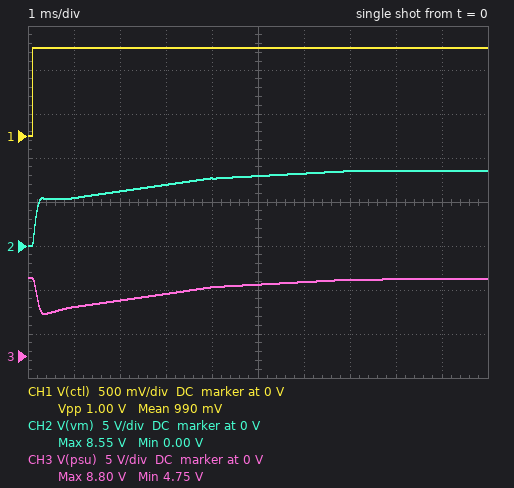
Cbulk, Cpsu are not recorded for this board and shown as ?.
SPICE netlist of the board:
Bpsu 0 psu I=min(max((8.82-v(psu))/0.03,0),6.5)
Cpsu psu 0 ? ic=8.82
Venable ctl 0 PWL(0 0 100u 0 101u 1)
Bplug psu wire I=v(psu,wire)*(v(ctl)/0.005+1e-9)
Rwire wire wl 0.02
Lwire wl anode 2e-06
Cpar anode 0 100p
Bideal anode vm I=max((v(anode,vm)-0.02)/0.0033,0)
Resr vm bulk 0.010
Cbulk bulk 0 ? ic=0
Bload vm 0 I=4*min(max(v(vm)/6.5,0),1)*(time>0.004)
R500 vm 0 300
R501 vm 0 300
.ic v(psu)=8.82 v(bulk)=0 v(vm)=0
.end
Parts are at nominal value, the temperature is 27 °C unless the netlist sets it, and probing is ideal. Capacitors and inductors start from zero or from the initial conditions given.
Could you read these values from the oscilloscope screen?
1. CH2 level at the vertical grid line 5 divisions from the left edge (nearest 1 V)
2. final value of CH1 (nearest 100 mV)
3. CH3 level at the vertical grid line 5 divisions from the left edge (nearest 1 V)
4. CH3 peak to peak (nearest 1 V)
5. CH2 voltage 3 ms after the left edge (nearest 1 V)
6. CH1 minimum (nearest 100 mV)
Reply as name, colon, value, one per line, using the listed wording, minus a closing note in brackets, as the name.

CH2 level at the vertical grid line 5 divisions from the left edge: 8 V
final value of CH1: 1.0 V
CH3 level at the vertical grid line 5 divisions from the left edge: 8 V
CH3 peak to peak: 4 V
CH2 voltage 3 ms after the left edge: 7 V
CH1 minimum: 0 V
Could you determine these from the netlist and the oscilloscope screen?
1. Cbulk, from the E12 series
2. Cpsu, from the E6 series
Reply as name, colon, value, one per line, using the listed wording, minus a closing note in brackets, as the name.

Cbulk, from the E12 series: 3.9 mF
Cpsu, from the E6 series: 4.7 mF
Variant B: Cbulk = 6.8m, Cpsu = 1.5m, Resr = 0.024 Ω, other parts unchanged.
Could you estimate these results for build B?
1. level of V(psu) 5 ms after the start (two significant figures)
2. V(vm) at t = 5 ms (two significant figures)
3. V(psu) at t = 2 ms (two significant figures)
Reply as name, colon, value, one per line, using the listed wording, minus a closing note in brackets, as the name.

level of V(psu) 5 ms after the start: 5.3 V
V(vm) at t = 5 ms: 5.1 V
V(psu) at t = 2 ms: 3.3 V
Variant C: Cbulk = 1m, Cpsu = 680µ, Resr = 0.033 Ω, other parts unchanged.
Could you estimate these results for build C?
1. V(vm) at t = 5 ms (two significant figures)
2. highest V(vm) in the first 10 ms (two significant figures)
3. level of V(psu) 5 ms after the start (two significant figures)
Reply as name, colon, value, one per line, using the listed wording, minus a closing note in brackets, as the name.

V(vm) at t = 5 ms: 8.6 V
highest V(vm) in the first 10 ms: 8.8 V
level of V(psu) 5 ms after the start: 8.7 V
